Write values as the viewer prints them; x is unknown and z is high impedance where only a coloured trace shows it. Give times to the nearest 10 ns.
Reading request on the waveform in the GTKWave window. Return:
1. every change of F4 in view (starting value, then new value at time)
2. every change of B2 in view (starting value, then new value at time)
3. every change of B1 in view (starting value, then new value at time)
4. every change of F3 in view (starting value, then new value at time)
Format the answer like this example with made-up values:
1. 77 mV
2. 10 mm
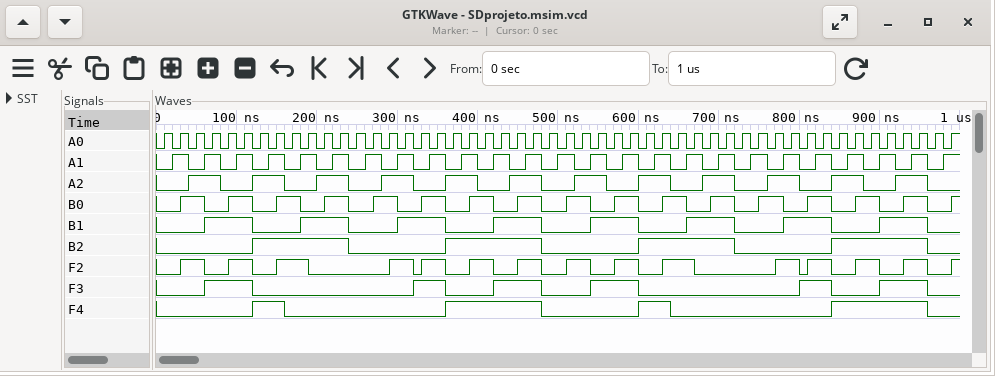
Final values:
1. 0, 1 at 120 ns, 0 at 160 ns, 1 at 360 ns, 0 at 480 ns, 1 at 600 ns, 0 at 640 ns, 1 at 840 ns, 0 at 960 ns
2. 0, 1 at 120 ns, 0 at 240 ns, 1 at 360 ns, 0 at 480 ns, 1 at 600 ns, 0 at 720 ns, 1 at 840 ns, 0 at 960 ns
3. 0, 1 at 60 ns, 0 at 120 ns, 1 at 180 ns, 0 at 240 ns, 1 at 300 ns, 0 at 360 ns, 1 at 420 ns, 0 at 480 ns, 1 at 540 ns, 0 at 600 ns, 1 at 660 ns, 0 at 720 ns, 1 at 780 ns, 0 at 840 ns, 1 at 900 ns, 0 at 960 ns
4. 0, 1 at 60 ns, 0 at 120 ns, 1 at 320 ns, 0 at 360 ns, 1 at 420 ns, 0 at 480 ns, 1 at 540 ns, 0 at 600 ns, 1 at 800 ns, 0 at 840 ns, 1 at 900 ns, 0 at 960 ns
